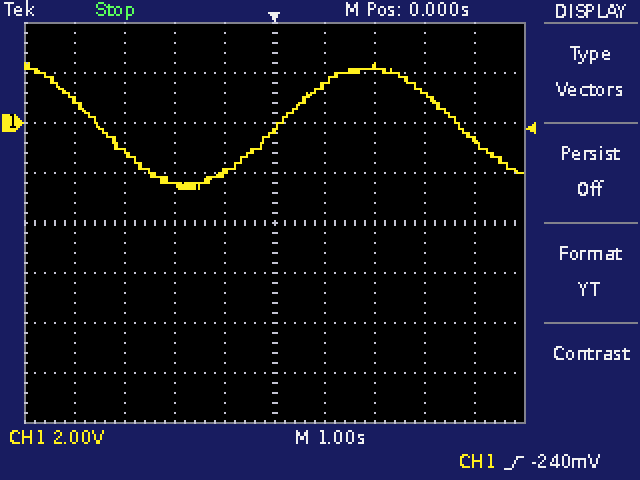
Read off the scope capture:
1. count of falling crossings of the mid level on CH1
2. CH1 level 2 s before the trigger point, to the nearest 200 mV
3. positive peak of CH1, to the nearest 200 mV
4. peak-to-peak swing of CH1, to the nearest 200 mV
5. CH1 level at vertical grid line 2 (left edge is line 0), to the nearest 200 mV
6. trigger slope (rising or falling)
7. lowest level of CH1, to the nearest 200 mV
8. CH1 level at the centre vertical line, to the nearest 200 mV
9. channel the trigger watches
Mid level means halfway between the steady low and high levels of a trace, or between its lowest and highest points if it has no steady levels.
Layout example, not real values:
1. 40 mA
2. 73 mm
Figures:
1. 2
2. -2.4 V
3. 2.4 V
4. 5.0 V
5. -1.2 V
6. rising
7. -2.6 V
8. -200 mV
9. CH1
